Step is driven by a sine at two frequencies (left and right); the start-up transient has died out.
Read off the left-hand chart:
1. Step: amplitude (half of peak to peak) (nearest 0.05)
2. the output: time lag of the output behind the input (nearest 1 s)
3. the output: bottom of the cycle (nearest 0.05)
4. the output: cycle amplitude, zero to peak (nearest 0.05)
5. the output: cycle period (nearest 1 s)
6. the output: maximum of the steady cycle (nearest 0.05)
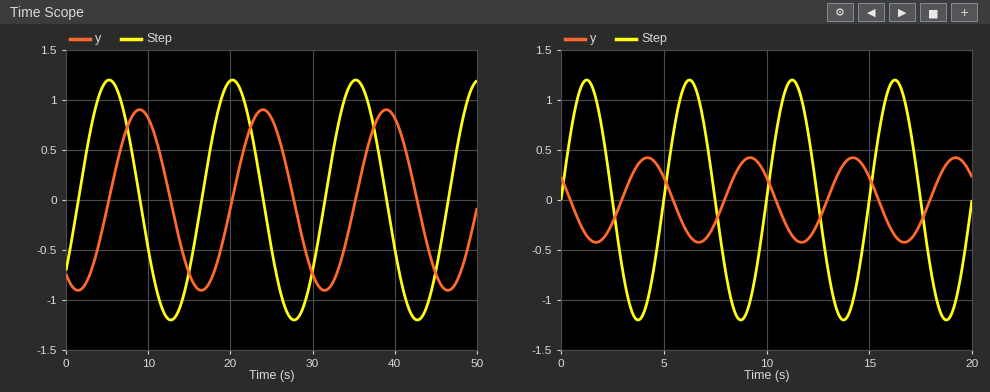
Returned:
1.20
4 s
-0.90
0.90
15 s
0.90
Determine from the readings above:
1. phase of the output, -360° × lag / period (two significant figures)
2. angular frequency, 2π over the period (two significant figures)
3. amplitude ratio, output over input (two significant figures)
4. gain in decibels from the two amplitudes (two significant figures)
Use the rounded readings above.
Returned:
-96°
0.42 rad/s
0.75
-2.5 dB
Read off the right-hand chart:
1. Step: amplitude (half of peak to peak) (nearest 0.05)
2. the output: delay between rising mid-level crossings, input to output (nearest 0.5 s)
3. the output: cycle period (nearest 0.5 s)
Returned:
1.20
3.0 s
5.0 s
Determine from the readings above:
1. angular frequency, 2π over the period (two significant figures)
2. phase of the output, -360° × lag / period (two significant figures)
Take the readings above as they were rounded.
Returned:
1.3 rad/s
-220°
